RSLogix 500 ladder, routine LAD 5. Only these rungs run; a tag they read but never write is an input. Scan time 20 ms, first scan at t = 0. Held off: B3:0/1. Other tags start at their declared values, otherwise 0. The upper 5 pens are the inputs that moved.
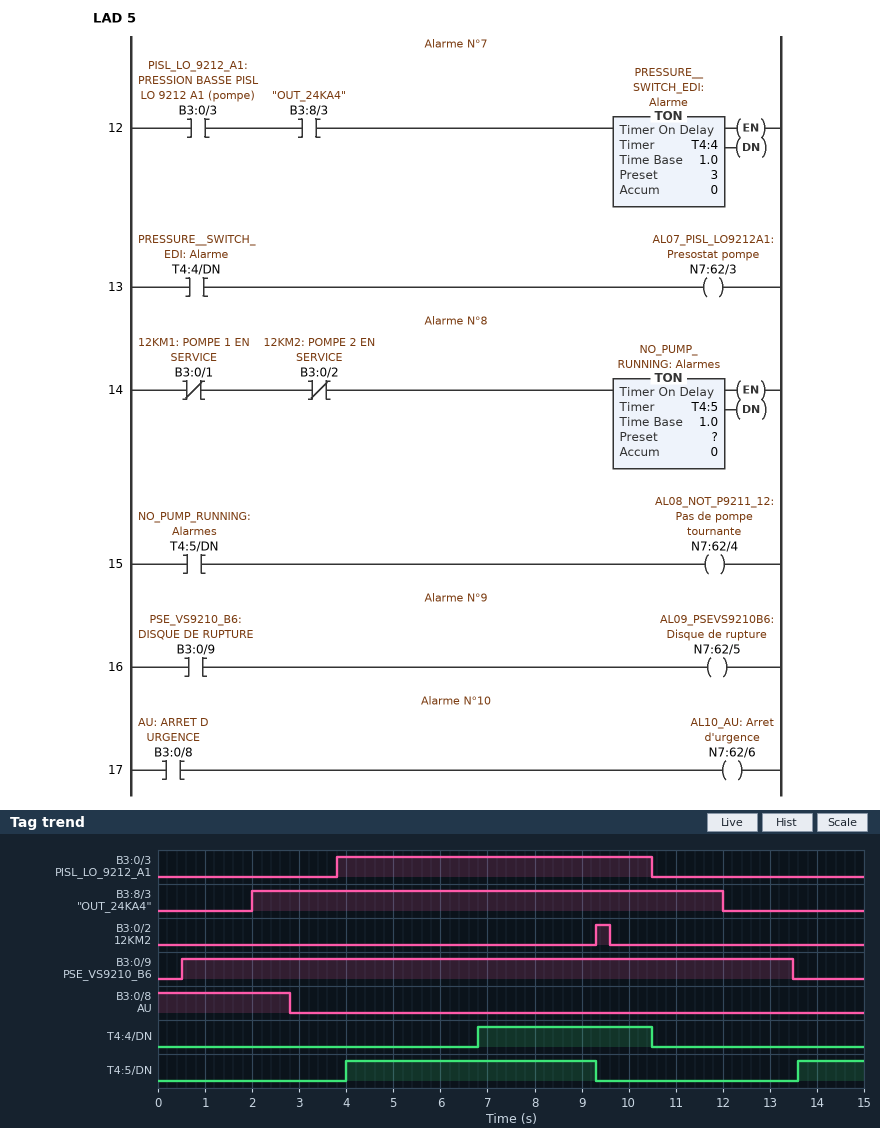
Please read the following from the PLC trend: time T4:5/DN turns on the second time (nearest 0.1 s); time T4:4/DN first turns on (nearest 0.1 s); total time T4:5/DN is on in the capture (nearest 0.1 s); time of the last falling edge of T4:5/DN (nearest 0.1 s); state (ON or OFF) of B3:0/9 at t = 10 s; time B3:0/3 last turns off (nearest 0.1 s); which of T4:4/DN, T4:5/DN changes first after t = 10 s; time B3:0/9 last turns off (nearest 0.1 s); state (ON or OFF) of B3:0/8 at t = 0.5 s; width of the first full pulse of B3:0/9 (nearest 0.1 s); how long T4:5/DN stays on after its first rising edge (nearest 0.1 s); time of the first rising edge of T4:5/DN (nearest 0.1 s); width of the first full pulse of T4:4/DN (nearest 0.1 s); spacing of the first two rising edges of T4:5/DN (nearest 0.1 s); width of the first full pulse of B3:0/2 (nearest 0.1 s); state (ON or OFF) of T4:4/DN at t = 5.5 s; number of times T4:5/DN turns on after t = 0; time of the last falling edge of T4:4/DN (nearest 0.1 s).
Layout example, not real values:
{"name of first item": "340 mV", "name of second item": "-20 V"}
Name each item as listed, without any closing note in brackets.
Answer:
{"time T4:5/DN turns on the second time": "13.6 s", "time T4:4/DN first turns on": "6.8 s", "total time T4:5/DN is on in the capture": "6.7 s", "time of the last falling edge of T4:5/DN": "9.3 s", "state (ON or OFF) of B3:0/9 at t = 10 s": "ON", "time B3:0/3 last turns off": "10.5 s", "which of T4:4/DN, T4:5/DN changes first after t = 10 s": "T4:4/DN", "time B3:0/9 last turns off": "13.5 s", "state (ON or OFF) of B3:0/8 at t = 0.5 s": "ON", "width of the first full pulse of B3:0/9": "13.0 s", "how long T4:5/DN stays on after its first rising edge": "5.3 s", "time of the first rising edge of T4:5/DN": "4.0 s", "width of the first full pulse of T4:4/DN": "3.7 s", "spacing of the first two rising edges of T4:5/DN": "9.6 s", "width of the first full pulse of B3:0/2": "0.3 s", "state (ON or OFF) of T4:4/DN at t = 5.5 s": "OFF", "number of times T4:5/DN turns on after t = 0": "2", "time of the last falling edge of T4:4/DN": "10.5 s"}
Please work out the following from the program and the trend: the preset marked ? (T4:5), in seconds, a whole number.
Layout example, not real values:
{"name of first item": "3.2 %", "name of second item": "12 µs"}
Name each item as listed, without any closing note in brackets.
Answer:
{"the preset marked ? (T4:5), in seconds, a whole number": "4 s"}
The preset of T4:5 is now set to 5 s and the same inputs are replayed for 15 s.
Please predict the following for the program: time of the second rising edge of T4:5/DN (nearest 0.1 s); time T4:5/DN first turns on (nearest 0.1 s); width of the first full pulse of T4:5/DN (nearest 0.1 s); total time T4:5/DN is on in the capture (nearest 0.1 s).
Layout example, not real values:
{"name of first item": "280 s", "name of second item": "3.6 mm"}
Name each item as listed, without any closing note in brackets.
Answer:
{"time of the second rising edge of T4:5/DN": "14.6 s", "time T4:5/DN first turns on": "5.0 s", "width of the first full pulse of T4:5/DN": "4.3 s", "total time T4:5/DN is on in the capture": "4.7 s"}
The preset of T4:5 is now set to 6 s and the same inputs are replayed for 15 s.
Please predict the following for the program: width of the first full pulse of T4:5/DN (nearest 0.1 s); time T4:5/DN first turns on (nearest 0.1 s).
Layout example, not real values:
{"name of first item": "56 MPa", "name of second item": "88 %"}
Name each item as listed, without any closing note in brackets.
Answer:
{"width of the first full pulse of T4:5/DN": "3.3 s", "time T4:5/DN first turns on": "6.0 s"}
